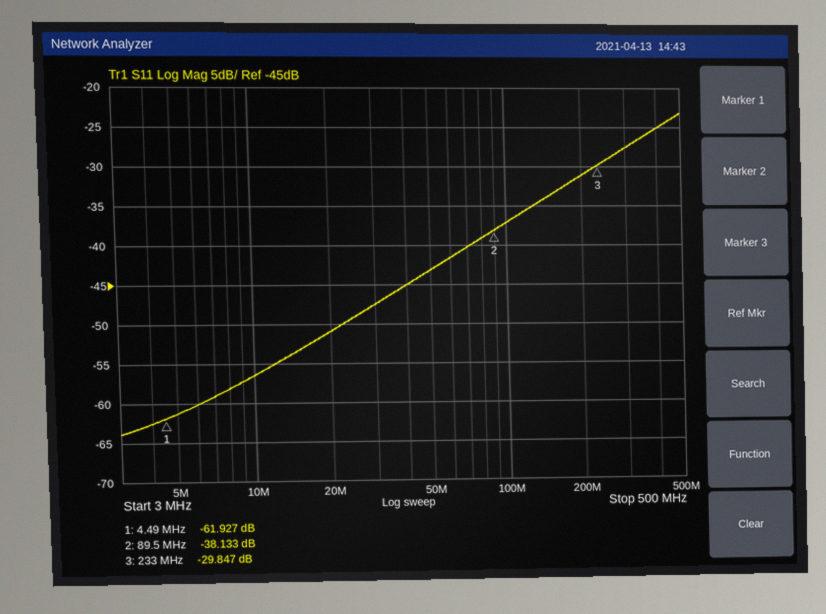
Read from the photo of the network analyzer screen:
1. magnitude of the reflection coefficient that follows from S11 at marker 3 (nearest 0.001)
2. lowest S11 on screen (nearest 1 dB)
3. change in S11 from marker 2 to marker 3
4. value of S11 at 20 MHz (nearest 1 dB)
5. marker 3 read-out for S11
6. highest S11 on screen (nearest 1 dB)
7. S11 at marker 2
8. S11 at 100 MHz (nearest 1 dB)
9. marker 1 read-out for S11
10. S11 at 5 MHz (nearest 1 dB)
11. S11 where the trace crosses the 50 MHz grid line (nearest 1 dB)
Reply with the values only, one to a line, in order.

0.032
-64 dB
8.286 dB
-51 dB
-29.847 dB
-23 dB
-38.133 dB
-37 dB
-61.927 dB
-61 dB
-43 dB
